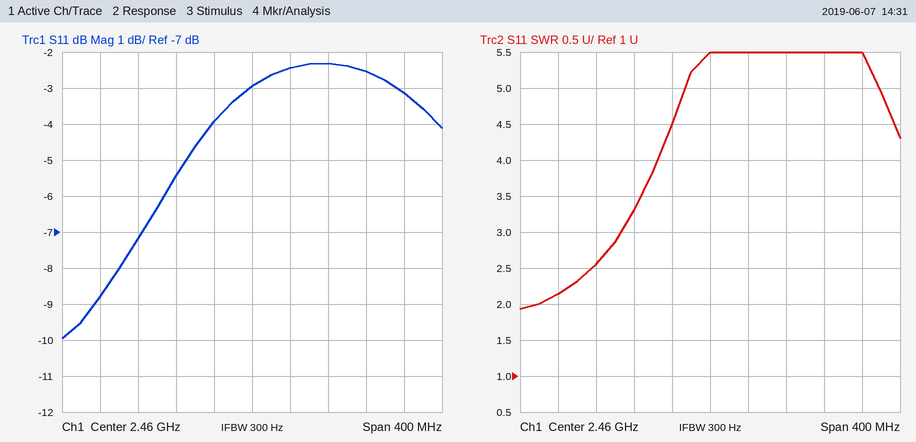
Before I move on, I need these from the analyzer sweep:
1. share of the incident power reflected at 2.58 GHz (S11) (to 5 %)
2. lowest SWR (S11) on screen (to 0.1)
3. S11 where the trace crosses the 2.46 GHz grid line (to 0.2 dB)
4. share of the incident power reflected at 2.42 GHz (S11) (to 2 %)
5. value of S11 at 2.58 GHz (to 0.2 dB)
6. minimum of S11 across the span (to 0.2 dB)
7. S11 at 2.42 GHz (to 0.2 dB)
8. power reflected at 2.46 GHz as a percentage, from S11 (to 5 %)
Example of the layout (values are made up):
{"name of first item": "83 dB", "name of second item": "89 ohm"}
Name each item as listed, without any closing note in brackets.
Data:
{"share of the incident power reflected at 2.58 GHz (S11)": "55 %", "lowest SWR (S11) on screen": "1.9", "S11 where the trace crosses the 2.46 GHz grid line": "-3.0 dB", "share of the incident power reflected at 2.42 GHz (S11)": "40 %", "value of S11 at 2.58 GHz": "-2.6 dB", "minimum of S11 across the span": "-10.0 dB", "S11 at 2.42 GHz": "-4.0 dB", "power reflected at 2.46 GHz as a percentage, from S11": "50 %"}
